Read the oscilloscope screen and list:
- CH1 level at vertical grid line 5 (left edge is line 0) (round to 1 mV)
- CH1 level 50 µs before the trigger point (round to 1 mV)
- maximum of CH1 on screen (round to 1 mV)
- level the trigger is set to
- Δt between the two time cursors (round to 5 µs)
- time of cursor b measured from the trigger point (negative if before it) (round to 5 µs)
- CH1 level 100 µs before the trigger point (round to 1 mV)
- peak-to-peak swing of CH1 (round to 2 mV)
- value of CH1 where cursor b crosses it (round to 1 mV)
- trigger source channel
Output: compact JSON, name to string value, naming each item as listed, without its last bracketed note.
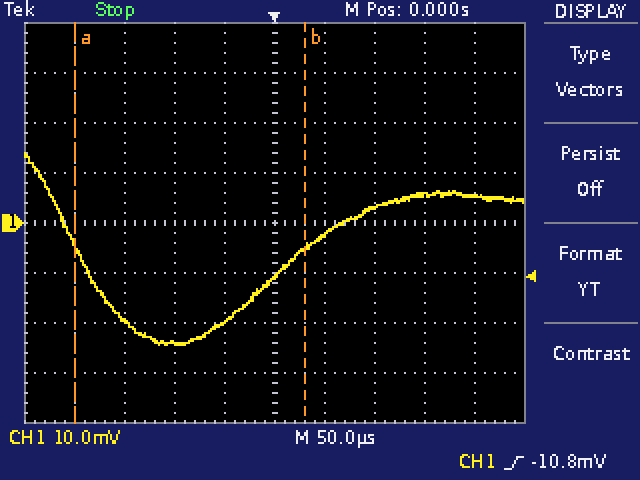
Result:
{"CH1 level at vertical grid line 5 (left edge is line 0)": "-11 mV", "CH1 level 50 µs before the trigger point": "-20 mV", "maximum of CH1 on screen": "14 mV", "level the trigger is set to": "-10.8 mV", "Δt between the two time cursors": "230 µs", "time of cursor b measured from the trigger point (negative if before it)": "+30 µs", "CH1 level 100 µs before the trigger point": "-24 mV", "peak-to-peak swing of CH1": "38 mV", "value of CH1 where cursor b crosses it": "-5 mV", "trigger source channel": "CH1"}
